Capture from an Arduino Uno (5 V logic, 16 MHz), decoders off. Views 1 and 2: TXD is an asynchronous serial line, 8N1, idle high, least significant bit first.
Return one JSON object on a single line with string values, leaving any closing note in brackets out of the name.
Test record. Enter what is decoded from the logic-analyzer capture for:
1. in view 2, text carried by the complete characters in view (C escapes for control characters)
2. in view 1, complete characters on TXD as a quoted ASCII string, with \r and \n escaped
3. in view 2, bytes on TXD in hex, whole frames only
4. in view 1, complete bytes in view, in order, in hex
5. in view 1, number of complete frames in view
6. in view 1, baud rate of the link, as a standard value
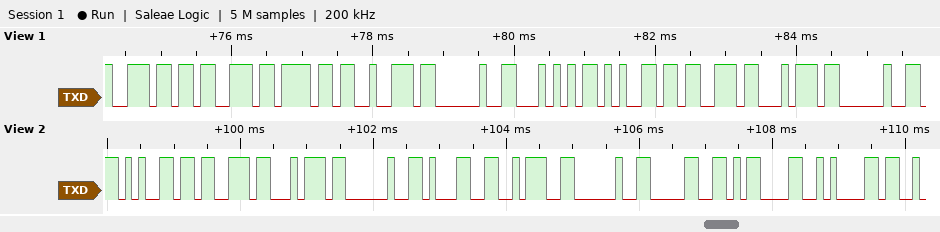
{"in view 2, text carried by the complete characters in view": "\"est 1: 0\\r\\n\"", "in view 1, complete characters on TXD as a quoted ASCII string, with \\r and \\n escaped": "\"nsor Test \"", "in view 2, bytes on TXD in hex, whole frames only": "65 73 74 20 31 3A 20 30 0D 0A", "in view 1, complete bytes in view, in order, in hex": "0x6E 0x73 0x6F 0x72 0x20 0x54 0x65 0x73 0x74 0x20", "in view 1, number of complete frames in view": "10", "in view 1, baud rate of the link, as a standard value": "9600 baud"}
